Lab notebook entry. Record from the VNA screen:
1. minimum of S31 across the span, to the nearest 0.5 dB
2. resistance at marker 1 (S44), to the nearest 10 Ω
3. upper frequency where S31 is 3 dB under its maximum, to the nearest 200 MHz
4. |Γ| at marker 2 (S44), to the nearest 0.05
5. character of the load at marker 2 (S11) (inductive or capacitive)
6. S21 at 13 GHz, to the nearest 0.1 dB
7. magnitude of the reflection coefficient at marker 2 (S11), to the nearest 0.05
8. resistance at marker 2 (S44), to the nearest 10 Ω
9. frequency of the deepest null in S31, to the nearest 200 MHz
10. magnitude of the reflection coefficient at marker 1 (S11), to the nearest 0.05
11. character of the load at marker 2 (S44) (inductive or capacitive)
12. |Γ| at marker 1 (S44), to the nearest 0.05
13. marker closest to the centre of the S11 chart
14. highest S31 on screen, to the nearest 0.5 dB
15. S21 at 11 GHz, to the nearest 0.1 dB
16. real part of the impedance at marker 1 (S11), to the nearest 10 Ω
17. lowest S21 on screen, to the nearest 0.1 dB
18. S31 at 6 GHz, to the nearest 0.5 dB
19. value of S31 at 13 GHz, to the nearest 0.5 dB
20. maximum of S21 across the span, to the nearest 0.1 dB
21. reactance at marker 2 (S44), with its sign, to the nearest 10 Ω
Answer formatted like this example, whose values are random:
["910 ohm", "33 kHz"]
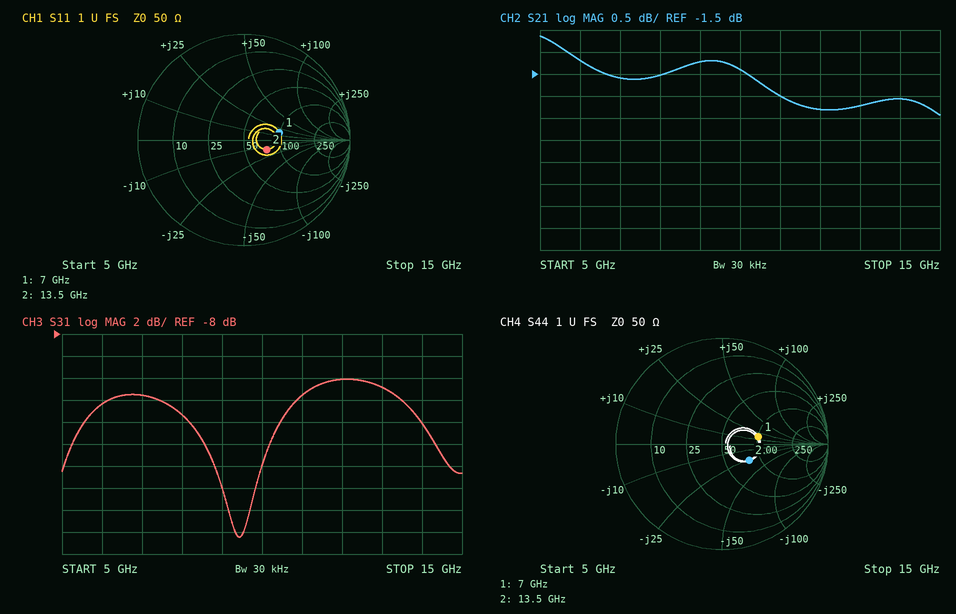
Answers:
["-26.5 dB", "100 Ω", "13.8 GHz", "0.30", "capacitive", "-2.2 dB", "0.25", "80 Ω", "9.4 GHz", "0.35", "capacitive", "0.35", "marker 2", "-12.0 dB", "-2.0 dB", "100 Ω", "-2.4 dB", "-14.5 dB", "-13.0 dB", "-0.6 dB", "-30 Ω"]
